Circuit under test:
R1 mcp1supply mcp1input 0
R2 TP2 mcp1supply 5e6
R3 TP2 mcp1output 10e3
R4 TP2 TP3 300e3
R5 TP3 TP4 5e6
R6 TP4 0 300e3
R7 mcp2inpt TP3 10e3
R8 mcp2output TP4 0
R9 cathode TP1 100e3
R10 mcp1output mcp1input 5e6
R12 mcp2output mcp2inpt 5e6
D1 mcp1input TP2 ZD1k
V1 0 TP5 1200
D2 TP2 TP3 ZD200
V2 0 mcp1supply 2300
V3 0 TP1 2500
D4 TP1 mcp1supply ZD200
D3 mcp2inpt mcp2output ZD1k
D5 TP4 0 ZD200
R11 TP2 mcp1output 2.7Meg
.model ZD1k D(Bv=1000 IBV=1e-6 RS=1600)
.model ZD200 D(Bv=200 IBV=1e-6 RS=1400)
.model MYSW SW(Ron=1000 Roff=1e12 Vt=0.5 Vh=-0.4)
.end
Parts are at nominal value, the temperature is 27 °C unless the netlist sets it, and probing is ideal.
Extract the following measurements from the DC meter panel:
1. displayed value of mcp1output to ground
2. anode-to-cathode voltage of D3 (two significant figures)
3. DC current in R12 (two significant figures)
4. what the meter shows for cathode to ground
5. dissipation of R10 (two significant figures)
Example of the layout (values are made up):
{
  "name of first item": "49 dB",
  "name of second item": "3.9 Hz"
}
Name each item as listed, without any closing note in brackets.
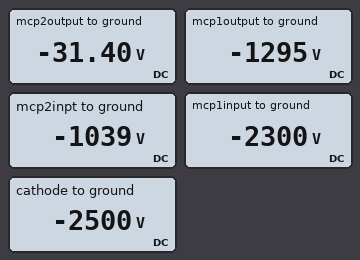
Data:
{
  "displayed value of mcp1output to ground": "-1295 V",
  "anode-to-cathode voltage of D3": "-1.0 kV",
  "DC current in R12": "200 µA",
  "what the meter shows for cathode to ground": "-2500 V",
  "dissipation of R10": "200 mW"
}
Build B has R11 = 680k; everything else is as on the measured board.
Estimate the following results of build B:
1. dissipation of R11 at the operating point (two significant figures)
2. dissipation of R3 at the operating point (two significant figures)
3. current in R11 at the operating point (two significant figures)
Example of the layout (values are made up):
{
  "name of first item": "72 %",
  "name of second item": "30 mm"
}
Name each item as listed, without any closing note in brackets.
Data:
{
  "dissipation of R11 at the operating point": "5.8 µW",
  "dissipation of R3 at the operating point": "390 µW",
  "current in R11 at the operating point": "2.9 µA"
}
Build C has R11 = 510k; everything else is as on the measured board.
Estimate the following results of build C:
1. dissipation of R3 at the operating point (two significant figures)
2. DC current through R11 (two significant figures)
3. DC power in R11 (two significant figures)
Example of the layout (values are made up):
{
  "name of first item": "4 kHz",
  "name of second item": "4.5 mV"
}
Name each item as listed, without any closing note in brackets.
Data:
{
  "dissipation of R3 at the operating point": "390 µW",
  "DC current through R11": "3.9 µA",
  "DC power in R11": "7.6 µW"
}
